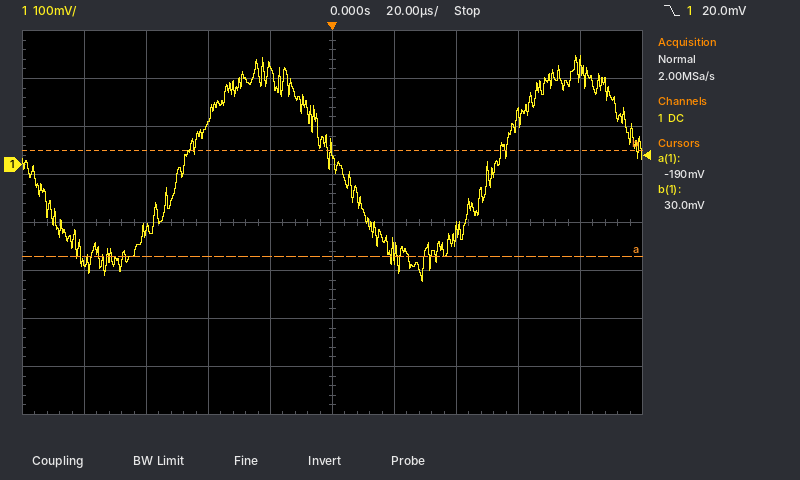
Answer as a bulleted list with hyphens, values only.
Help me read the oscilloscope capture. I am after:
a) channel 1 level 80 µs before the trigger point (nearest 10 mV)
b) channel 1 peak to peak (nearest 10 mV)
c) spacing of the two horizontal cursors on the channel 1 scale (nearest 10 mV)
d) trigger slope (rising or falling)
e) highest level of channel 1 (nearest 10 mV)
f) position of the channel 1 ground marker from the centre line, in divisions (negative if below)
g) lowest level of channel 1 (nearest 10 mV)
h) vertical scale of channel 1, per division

- -200 mV
- 470 mV
- 220 mV
- falling
- 230 mV
- +1.2 div
- -240 mV
- 100 mV
